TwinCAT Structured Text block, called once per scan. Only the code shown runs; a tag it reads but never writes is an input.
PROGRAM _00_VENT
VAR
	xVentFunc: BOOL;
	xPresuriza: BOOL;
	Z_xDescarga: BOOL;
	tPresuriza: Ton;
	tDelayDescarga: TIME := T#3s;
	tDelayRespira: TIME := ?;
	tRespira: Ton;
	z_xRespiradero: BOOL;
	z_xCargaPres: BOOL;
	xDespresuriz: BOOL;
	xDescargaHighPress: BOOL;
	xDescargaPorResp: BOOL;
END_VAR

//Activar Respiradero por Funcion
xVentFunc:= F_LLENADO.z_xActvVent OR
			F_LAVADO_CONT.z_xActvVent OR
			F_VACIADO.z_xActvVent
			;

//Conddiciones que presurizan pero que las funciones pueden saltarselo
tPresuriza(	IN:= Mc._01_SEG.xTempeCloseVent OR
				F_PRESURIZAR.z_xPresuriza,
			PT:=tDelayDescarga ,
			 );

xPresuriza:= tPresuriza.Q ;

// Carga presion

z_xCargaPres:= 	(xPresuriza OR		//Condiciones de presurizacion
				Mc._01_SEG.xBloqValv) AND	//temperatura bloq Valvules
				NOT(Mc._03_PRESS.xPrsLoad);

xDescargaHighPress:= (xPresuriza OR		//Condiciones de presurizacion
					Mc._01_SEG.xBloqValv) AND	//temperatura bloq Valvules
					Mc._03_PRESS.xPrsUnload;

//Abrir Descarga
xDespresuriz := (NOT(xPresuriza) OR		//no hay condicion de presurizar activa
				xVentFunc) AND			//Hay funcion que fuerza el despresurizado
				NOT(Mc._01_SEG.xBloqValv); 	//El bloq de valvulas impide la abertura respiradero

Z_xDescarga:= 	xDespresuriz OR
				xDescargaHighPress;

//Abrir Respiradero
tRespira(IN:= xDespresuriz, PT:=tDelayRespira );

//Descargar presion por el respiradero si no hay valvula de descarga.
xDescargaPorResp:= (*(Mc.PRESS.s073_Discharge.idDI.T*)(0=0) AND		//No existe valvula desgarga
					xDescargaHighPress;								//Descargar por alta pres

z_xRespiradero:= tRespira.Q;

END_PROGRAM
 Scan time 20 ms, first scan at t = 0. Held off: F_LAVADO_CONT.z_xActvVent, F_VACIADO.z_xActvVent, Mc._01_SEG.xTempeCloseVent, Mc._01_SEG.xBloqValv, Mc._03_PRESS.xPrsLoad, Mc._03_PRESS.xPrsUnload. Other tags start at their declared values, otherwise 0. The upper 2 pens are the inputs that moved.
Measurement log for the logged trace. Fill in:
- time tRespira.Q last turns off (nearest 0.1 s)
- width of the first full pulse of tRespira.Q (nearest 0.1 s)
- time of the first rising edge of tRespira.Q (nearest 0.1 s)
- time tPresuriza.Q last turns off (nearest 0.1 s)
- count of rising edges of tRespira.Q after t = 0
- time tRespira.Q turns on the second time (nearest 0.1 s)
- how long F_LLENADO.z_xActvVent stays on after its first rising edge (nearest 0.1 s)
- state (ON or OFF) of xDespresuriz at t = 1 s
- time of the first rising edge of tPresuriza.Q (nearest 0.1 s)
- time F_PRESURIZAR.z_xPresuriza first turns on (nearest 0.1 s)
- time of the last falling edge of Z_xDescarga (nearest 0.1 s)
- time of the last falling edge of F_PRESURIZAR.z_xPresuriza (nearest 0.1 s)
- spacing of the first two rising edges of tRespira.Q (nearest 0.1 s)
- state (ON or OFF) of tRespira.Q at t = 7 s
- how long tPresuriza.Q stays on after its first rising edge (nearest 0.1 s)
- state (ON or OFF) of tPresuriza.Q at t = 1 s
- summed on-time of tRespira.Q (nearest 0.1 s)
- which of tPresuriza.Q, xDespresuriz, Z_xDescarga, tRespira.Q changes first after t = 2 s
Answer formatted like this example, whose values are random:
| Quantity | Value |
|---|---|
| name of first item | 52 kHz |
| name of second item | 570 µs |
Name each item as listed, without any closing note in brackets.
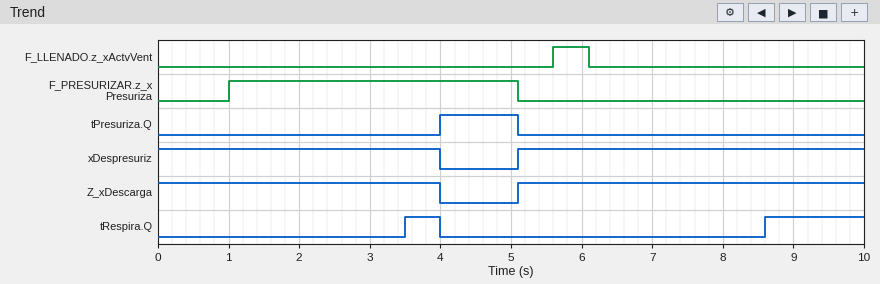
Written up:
| Quantity | Value |
|---|---|
| time tRespira.Q last turns off | 4.0 s |
| width of the first full pulse of tRespira.Q | 0.5 s |
| time of the first rising edge of tRespira.Q | 3.5 s |
| time tPresuriza.Q last turns off | 5.1 s |
| count of rising edges of tRespira.Q after t = 0 | 2 |
| time tRespira.Q turns on the second time | 8.6 s |
| how long F_LLENADO.z_xActvVent stays on after its first rising edge | 0.5 s |
| state (ON or OFF) of xDespresuriz at t = 1 s | ON |
| time of the first rising edge of tPresuriza.Q | 4.0 s |
| time F_PRESURIZAR.z_xPresuriza first turns on | 1.0 s |
| time of the last falling edge of Z_xDescarga | 4.0 s |
| time of the last falling edge of F_PRESURIZAR.z_xPresuriza | 5.1 s |
| spacing of the first two rising edges of tRespira.Q | 5.1 s |
| state (ON or OFF) of tRespira.Q at t = 7 s | OFF |
| how long tPresuriza.Q stays on after its first rising edge | 1.1 s |
| state (ON or OFF) of tPresuriza.Q at t = 1 s | OFF |
| summed on-time of tRespira.Q | 1.9 s |
| which of tPresuriza.Q, xDespresuriz, Z_xDescarga, tRespira.Q changes first after t = 2 s | tRespira.Q |
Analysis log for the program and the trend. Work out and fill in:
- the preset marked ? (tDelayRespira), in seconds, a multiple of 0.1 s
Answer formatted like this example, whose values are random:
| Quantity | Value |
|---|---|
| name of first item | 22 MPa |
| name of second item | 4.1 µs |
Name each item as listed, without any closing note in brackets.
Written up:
| Quantity | Value |
|---|---|
| the preset marked ? (tDelayRespira), in seconds, a multiple of 0.1 s | 3.5 s |
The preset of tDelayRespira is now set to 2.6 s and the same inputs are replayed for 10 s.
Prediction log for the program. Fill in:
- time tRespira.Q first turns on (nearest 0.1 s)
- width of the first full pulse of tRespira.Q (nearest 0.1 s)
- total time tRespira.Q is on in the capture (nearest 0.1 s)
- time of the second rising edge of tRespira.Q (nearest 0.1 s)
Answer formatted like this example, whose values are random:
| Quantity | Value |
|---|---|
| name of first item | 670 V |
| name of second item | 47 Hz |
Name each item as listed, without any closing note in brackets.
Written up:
| Quantity | Value |
|---|---|
| time tRespira.Q first turns on | 2.6 s |
| width of the first full pulse of tRespira.Q | 1.4 s |
| total time tRespira.Q is on in the capture | 3.7 s |
| time of the second rising edge of tRespira.Q | 7.7 s |
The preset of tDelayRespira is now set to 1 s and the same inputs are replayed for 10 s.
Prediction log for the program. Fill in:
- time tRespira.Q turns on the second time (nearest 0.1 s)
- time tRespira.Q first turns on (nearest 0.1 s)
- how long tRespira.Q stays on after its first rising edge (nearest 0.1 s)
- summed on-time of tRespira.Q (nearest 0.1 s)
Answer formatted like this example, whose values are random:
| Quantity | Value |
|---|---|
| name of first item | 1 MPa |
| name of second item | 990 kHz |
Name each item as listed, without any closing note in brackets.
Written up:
| Quantity | Value |
|---|---|
| time tRespira.Q turns on the second time | 6.1 s |
| time tRespira.Q first turns on | 1.0 s |
| how long tRespira.Q stays on after its first rising edge | 3.0 s |
| summed on-time of tRespira.Q | 6.9 s |
